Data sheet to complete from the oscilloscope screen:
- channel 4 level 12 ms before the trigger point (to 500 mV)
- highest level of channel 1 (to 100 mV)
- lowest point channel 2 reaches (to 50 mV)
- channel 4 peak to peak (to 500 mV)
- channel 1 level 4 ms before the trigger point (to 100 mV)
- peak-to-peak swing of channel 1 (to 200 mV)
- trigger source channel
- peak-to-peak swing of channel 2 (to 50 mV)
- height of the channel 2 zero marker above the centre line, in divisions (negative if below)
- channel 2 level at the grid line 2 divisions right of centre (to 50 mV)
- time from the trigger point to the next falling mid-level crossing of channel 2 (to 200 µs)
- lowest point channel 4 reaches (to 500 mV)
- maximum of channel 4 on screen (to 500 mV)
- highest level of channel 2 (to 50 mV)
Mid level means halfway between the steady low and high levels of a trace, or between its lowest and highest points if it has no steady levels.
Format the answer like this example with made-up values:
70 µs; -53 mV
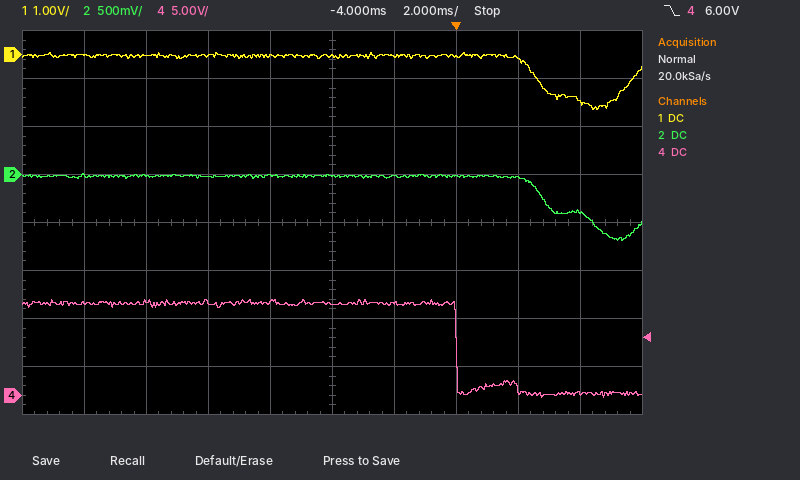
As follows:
9.5 V; 0.0 V; -700 mV; 10.0 V; 0.0 V; 1.2 V; channel 4; 700 mV; +1.0 div; 0 mV; 3.0 ms; 0.0 V; 10.0 V; 0 mV
